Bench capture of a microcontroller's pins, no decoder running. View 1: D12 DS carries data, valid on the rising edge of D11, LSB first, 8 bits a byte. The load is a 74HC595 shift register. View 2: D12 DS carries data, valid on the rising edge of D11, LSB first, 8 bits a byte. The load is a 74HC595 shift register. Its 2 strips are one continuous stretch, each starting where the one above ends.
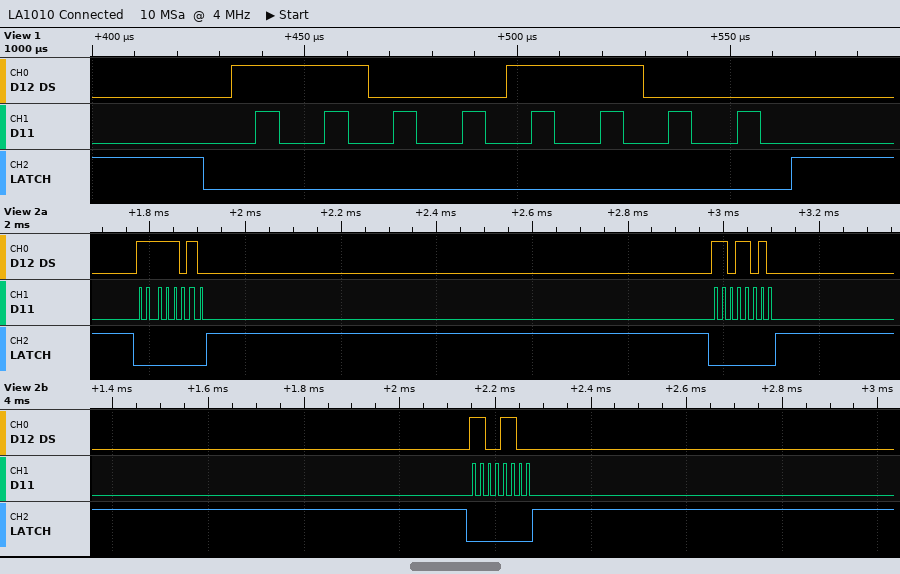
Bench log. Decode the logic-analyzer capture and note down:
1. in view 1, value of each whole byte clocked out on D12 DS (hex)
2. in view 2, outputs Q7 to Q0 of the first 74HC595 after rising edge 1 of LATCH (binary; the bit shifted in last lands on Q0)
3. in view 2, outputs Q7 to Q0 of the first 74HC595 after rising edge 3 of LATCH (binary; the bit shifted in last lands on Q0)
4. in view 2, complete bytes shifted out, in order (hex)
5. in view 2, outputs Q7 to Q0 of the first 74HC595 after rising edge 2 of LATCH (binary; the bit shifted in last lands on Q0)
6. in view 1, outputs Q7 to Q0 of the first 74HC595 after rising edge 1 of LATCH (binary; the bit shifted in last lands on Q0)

33
11111010
11001100
5F 5B 33
11011010
11001100
